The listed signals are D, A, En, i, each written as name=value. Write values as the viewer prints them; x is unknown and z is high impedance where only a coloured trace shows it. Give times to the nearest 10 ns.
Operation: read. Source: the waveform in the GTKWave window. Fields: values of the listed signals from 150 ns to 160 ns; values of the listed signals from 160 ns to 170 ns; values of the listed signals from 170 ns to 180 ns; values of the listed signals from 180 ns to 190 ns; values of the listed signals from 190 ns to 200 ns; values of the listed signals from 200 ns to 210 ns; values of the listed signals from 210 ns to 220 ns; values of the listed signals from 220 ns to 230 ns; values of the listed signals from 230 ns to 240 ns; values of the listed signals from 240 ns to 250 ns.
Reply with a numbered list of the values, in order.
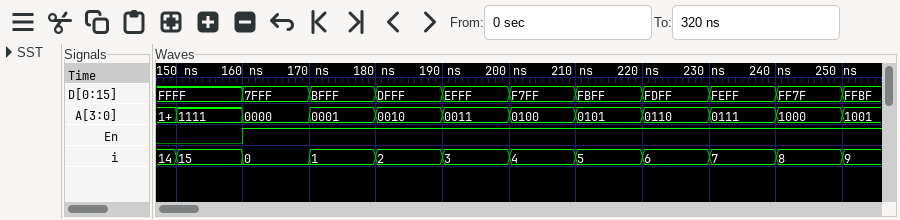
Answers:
1. D=FFFF, A=1111, En=0, i=15
2. D=7FFF, A=0000, En=1, i=0
3. D=BFFF, A=0001, En=1, i=1
4. D=DFFF, A=0010, En=1, i=2
5. D=EFFF, A=0011, En=1, i=3
6. D=F7FF, A=0100, En=1, i=4
7. D=FBFF, A=0101, En=1, i=5
8. D=FDFF, A=0110, En=1, i=6
9. D=FEFF, A=0111, En=1, i=7
10. D=FF7F, A=1000, En=1, i=8
